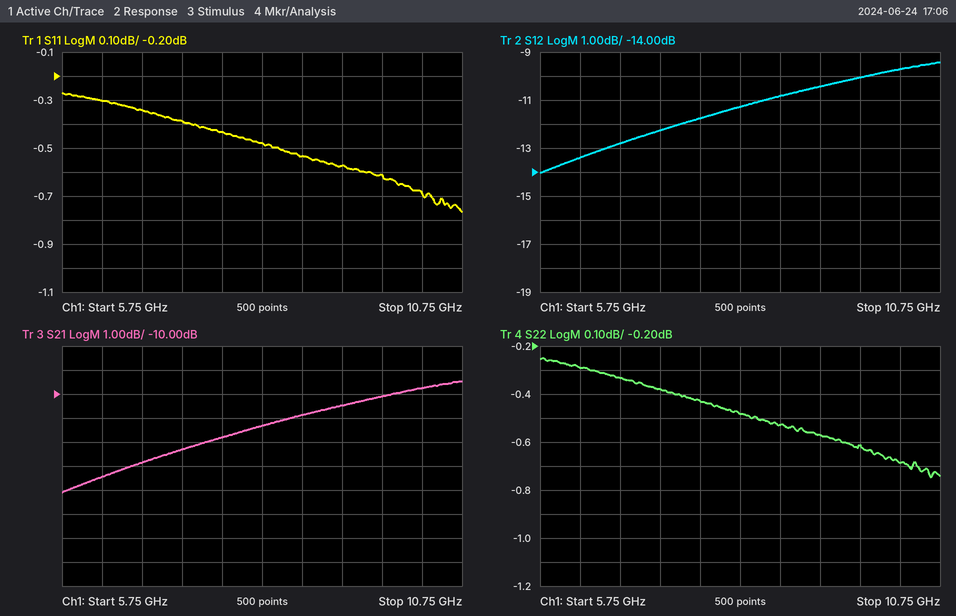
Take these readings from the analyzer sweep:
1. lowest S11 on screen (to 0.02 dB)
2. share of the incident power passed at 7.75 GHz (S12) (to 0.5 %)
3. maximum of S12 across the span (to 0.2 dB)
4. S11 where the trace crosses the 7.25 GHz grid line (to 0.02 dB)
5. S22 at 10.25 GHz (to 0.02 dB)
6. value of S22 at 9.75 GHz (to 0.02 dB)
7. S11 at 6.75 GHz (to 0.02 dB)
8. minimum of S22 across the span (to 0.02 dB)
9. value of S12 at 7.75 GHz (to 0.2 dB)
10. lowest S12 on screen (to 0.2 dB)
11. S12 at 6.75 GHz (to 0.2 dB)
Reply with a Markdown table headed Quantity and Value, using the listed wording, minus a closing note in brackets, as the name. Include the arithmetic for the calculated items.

| Quantity | Value |
|---|---|
| lowest S11 on screen | -0.76 dB |
| share of the incident power passed at 7.75 GHz (S12) | 10^(-11.8/10) ≈ 6.61 %, so 6.5 % to the nearest 0.5 % |
| maximum of S12 across the span | -9.4 dB |
| S11 where the trace crosses the 7.25 GHz grid line | -0.38 dB |
| S22 at 10.25 GHz | -0.68 dB |
| value of S22 at 9.75 GHz | -0.62 dB |
| S11 at 6.75 GHz | -0.34 dB |
| minimum of S22 across the span | -0.74 dB |
| value of S12 at 7.75 GHz | -11.8 dB |
| lowest S12 on screen | -14.0 dB |
| S12 at 6.75 GHz | -12.8 dB |
